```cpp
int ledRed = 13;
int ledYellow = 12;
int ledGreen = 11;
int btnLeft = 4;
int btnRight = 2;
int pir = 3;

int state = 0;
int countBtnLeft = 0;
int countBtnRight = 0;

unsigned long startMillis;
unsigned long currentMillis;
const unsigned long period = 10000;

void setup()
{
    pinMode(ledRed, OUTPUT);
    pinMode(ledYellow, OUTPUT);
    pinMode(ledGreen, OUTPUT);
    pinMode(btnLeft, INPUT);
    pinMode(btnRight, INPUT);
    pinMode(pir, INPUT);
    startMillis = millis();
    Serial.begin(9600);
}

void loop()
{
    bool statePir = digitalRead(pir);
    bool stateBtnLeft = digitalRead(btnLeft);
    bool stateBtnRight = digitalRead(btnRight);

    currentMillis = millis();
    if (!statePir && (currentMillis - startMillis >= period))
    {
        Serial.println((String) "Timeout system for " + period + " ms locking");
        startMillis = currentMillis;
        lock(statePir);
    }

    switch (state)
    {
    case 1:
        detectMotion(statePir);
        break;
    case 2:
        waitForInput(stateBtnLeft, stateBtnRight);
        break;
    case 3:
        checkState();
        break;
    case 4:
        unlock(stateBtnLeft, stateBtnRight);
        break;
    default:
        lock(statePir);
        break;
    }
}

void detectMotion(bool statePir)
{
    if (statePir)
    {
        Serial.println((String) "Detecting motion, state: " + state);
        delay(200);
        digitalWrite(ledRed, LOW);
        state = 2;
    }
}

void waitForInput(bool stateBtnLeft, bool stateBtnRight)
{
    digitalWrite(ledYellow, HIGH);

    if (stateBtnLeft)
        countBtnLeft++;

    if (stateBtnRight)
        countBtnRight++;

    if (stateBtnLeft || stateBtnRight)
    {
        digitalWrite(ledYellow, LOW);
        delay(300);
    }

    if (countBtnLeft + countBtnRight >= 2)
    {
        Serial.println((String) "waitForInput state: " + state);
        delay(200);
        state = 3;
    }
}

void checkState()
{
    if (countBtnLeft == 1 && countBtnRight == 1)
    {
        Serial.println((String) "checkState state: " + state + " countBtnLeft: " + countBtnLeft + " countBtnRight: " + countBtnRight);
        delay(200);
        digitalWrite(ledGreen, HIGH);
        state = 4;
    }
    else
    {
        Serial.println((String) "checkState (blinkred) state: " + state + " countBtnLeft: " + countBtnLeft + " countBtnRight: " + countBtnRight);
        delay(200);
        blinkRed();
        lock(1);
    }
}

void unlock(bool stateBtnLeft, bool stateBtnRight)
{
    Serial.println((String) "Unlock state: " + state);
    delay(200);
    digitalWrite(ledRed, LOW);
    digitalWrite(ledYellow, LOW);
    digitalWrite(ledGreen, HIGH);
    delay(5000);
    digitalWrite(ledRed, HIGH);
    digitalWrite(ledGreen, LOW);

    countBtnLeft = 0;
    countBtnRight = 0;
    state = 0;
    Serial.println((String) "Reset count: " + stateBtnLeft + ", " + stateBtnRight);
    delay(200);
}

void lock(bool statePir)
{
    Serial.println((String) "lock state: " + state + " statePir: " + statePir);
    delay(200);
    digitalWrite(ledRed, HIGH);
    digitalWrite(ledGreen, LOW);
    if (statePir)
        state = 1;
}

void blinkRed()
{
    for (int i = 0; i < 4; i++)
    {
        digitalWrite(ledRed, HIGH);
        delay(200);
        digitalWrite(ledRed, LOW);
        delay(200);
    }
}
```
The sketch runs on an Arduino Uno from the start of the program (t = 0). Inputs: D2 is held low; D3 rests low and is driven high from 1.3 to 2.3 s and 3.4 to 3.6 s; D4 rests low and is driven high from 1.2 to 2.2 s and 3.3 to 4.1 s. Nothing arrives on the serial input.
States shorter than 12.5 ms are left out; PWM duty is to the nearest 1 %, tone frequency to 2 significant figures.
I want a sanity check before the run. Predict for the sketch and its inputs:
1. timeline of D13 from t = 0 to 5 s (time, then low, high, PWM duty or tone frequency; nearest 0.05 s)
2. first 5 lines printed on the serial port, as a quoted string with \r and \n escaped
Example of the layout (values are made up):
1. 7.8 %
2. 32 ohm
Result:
1. 0 s low; 0.2 s high; 1.8 s low; 2.8 s high; 3 s low; 3.2 s high; 3.4 s low; 3.6 s high; 3.8 s low; 4 s high; 4.2 s low; 4.6 s high
2. "lock state: 0 statePir: 0\r\nlock state: 0 statePir: 0\r\nlock state: 0 statePir: 0\r\nlock state: 0 statePir: 0\r\nlock state: 0 statePir: 0\r\n"
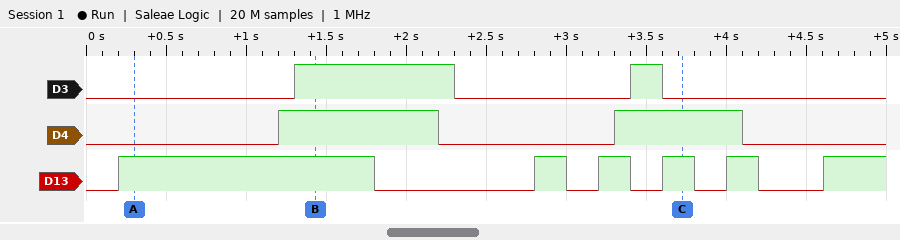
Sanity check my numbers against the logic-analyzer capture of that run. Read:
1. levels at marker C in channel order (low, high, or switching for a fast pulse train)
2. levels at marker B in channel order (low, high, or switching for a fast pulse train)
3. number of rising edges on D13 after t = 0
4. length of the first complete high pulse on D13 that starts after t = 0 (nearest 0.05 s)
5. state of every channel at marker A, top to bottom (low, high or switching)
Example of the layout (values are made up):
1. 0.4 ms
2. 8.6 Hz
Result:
1. D3 low, D4 high, D13 high
2. D3 high, D4 high, D13 high
3. 6
4. 1.60 s
5. D3 low, D4 low, D13 high
